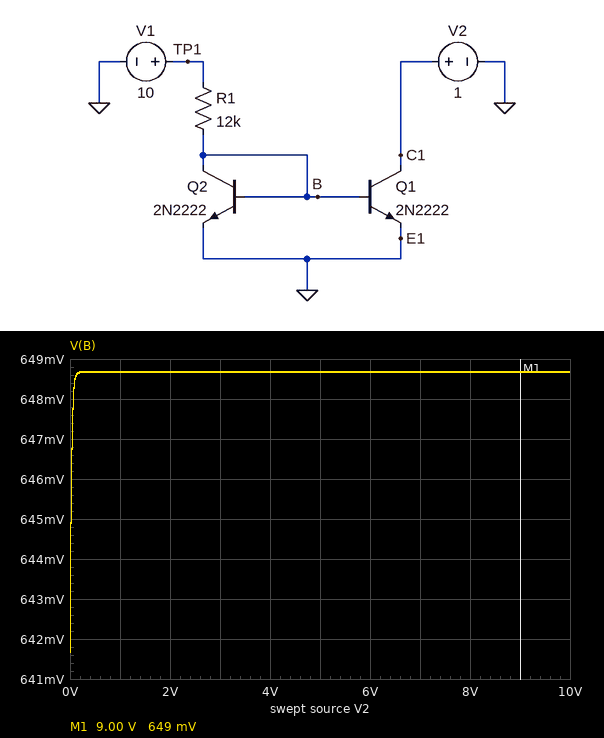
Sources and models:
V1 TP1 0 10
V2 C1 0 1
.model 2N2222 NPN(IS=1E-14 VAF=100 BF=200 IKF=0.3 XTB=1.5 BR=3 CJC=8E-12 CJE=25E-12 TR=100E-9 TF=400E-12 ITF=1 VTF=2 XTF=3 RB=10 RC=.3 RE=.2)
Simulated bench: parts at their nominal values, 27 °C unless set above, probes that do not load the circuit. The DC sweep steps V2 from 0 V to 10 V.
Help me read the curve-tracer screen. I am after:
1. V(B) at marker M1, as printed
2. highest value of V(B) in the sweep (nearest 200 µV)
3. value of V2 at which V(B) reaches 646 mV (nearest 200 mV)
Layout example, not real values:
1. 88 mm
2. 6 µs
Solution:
1. 649 mV
2. 648.6 mV
3. 0 V
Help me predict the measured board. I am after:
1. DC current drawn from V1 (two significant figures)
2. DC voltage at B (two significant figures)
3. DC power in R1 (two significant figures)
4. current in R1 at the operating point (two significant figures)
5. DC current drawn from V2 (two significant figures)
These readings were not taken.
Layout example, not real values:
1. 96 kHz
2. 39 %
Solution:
1. 780 µA
2. 650 mV
3. 7.3 mW
4. 780 µA
5. 770 µA
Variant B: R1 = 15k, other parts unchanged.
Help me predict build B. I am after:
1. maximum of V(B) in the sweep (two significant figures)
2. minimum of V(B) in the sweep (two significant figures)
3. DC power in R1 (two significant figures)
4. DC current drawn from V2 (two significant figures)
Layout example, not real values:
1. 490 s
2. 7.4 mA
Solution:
1. 640 mV
2. 640 mV
3. 5.8 mW
4. 620 µA
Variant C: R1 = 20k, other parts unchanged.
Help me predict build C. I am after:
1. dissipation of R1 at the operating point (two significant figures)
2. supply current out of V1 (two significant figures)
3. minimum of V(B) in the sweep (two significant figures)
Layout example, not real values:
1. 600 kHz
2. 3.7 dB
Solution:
1. 4.4 mW
2. 470 µA
3. 630 mV
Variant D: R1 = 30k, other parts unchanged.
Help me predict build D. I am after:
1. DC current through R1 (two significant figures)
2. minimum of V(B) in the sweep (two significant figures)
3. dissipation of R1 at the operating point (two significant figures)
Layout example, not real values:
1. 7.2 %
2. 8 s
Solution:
1. 310 µA
2. 620 mV
3. 2.9 mW
